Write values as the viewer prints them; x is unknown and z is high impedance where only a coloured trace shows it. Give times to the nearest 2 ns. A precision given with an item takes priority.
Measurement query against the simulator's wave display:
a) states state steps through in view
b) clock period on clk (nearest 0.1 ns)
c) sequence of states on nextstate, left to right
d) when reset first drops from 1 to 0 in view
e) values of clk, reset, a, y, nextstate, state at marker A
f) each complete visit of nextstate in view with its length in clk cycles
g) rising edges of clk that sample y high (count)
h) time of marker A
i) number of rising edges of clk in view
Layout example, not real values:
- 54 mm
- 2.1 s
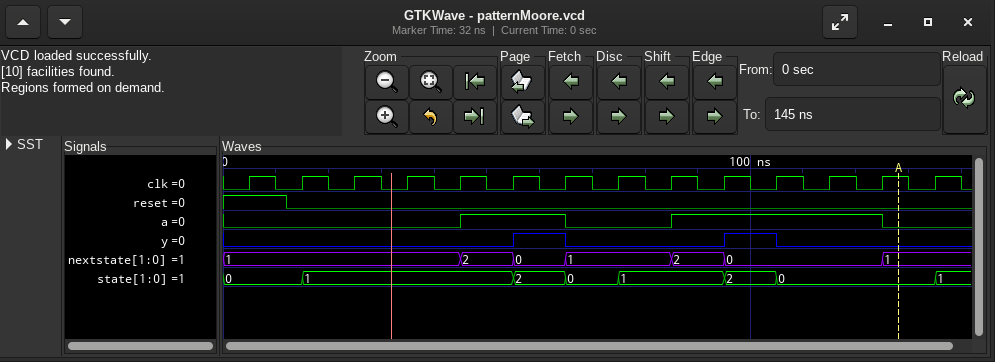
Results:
- 0, 1, 2, 0, 1, 2, 0, 1
- 10 ns
- 1, 2, 0, 1, 2, 0, 1
- 12 ns
- clk=1, reset=0, a=0, y=0, nextstate=1, state=0
- 2: 1, 0: 1, 1: 2, 2: 1, 0: 3
- 2
- 128 ns
- 14
